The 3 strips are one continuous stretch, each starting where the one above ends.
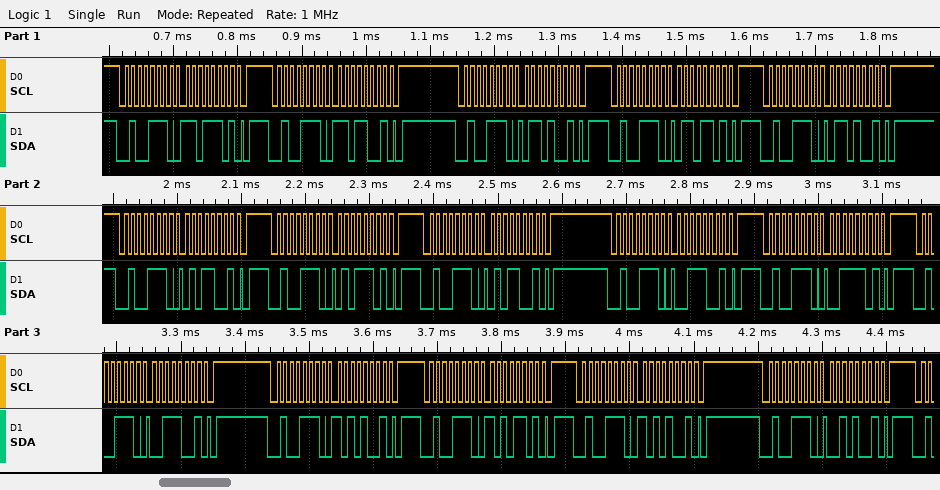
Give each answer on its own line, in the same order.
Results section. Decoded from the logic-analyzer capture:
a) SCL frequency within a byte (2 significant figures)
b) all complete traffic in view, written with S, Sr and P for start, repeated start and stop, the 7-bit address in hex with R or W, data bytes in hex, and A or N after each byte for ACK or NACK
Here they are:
100 kHz
S 27W A DD A P S 27W A D9 A P S 27W A 69 A P S 27W A 6D A P S 27W A 69 A P S 27W A 59 A P S 27W A 5D A P S 27W A 59 A P S 27W A 39 A P S 27W A 3D A P S 27W A 39 A P S 27W A A9 A P S 27W A AD A P S 27W A A9 A P S 27W A 29 A P
